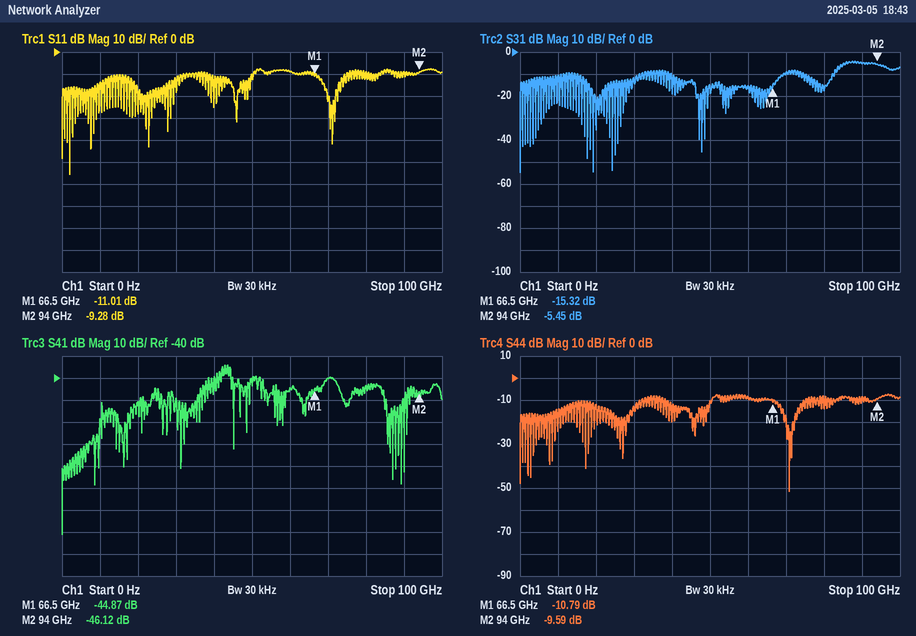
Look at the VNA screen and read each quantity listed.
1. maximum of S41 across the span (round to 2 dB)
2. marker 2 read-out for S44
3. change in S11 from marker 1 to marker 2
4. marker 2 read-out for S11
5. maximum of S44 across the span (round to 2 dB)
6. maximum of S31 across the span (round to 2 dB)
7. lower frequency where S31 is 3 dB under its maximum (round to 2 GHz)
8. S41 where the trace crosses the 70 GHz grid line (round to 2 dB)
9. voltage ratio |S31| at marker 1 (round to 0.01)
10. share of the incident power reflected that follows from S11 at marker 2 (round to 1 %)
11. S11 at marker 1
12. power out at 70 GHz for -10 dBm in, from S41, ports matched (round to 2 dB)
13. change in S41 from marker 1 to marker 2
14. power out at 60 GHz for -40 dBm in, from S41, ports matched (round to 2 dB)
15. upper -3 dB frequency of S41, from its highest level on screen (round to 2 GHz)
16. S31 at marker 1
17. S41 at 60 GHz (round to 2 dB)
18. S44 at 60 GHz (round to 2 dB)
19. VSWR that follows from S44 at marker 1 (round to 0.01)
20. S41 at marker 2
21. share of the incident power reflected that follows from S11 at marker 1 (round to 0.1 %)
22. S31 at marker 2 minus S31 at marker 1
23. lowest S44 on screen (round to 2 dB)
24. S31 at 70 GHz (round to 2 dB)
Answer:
-34 dB
-9.59 dB
1.73 dB
-9.28 dB
-8 dB
-4 dB
84 GHz
-40 dB
0.17
12 %
-11.01 dB
-50 dBm
-1.25 dB
-84 dBm
44 GHz
-15.32 dB
-44 dB
-8 dB
1.81
-46.12 dB
7.9 %
9.87 dB
-52 dB
-10 dB
